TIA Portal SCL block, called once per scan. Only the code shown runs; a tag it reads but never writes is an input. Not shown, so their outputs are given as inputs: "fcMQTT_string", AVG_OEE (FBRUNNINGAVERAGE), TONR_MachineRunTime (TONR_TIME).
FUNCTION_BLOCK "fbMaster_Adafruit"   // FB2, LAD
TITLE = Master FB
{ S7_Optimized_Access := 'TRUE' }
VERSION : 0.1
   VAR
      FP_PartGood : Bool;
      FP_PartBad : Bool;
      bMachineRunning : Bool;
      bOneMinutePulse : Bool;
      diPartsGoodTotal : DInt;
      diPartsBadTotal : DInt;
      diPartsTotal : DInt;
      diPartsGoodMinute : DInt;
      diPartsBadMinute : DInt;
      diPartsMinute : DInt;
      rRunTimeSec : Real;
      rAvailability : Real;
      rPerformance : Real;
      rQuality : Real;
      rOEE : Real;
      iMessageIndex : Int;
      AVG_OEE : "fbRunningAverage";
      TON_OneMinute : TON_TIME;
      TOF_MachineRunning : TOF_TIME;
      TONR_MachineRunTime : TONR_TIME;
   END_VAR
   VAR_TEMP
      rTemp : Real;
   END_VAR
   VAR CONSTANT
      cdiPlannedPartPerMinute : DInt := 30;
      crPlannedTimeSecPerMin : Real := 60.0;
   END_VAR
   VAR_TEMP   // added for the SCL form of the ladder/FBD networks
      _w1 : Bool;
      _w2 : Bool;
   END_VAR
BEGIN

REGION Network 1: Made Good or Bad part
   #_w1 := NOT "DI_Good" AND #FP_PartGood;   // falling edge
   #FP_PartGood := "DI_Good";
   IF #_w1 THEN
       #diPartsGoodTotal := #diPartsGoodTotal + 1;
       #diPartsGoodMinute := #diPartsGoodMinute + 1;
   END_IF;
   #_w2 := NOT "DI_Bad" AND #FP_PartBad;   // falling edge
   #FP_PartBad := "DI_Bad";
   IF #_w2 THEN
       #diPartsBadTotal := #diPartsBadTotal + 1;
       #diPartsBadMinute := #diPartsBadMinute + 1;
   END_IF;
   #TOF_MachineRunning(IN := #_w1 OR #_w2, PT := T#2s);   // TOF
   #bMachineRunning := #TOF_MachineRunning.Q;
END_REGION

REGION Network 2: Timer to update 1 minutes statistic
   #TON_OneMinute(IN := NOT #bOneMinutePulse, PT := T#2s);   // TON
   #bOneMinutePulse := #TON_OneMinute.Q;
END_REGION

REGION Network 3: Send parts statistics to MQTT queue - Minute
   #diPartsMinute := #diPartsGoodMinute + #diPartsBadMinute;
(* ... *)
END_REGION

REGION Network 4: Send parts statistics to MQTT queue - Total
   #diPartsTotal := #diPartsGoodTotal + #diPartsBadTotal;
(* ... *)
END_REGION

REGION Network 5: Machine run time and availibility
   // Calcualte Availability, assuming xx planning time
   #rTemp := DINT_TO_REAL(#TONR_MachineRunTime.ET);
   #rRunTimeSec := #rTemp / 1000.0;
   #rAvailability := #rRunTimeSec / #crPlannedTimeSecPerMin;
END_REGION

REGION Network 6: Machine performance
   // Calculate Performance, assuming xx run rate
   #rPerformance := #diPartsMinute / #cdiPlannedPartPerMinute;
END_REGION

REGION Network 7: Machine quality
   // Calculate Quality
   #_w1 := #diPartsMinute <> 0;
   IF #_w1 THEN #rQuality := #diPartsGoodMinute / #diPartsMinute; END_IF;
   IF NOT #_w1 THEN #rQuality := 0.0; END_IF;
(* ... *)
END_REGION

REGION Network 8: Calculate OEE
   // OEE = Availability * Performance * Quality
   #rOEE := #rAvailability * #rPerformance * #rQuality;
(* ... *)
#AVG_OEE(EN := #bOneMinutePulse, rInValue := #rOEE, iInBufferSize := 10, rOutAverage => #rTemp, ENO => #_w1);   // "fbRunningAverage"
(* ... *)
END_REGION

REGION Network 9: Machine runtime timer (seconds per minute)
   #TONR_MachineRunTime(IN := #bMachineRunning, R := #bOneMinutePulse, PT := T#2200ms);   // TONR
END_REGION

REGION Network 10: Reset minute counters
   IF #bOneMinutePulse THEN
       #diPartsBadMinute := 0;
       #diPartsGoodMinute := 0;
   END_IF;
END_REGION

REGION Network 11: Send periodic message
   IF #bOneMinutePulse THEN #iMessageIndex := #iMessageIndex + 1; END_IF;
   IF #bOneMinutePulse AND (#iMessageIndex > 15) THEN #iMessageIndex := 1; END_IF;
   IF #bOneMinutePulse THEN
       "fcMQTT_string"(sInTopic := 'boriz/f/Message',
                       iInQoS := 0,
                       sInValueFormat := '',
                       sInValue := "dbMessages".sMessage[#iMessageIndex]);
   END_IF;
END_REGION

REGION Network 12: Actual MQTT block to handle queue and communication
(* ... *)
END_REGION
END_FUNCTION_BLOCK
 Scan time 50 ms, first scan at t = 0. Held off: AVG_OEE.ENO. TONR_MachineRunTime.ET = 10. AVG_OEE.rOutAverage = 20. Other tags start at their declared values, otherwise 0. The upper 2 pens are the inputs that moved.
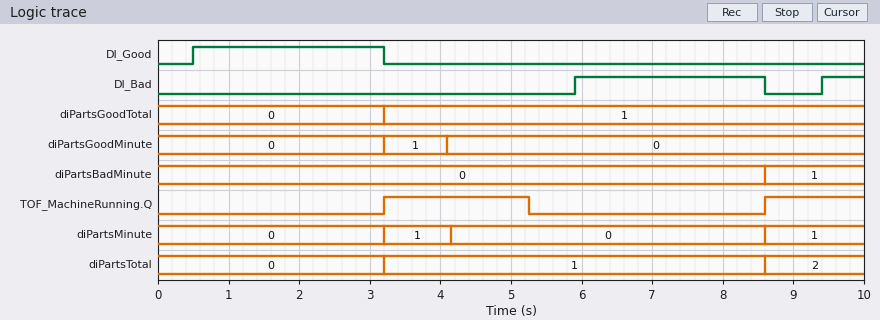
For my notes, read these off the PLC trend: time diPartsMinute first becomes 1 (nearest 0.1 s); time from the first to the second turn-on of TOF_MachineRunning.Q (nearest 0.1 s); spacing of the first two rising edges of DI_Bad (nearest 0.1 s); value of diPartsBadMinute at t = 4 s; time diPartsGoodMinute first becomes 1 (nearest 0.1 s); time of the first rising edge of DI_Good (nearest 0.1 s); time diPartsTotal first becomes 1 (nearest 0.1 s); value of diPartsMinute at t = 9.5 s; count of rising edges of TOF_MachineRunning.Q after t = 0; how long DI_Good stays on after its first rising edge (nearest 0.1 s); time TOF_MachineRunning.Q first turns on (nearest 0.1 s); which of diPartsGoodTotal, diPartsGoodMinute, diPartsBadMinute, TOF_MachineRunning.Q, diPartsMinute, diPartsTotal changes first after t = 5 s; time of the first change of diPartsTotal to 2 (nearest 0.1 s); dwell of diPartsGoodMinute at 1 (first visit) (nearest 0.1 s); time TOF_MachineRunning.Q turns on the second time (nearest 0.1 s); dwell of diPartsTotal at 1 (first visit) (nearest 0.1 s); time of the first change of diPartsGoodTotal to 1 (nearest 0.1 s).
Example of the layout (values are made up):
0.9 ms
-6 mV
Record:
3.2 s
5.4 s
3.5 s
0
3.2 s
0.5 s
3.2 s
1
2
2.7 s
3.2 s
TOF_MachineRunning.Q
8.6 s
0.9 s
8.6 s
5.4 s
3.2 s
